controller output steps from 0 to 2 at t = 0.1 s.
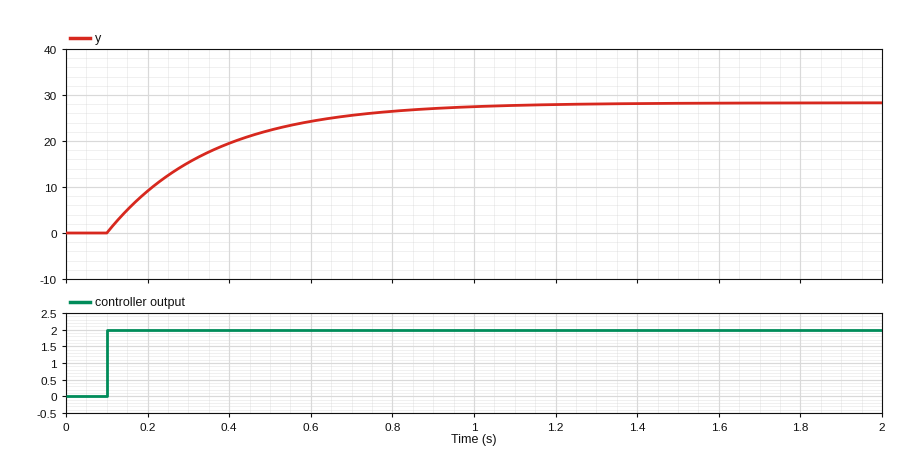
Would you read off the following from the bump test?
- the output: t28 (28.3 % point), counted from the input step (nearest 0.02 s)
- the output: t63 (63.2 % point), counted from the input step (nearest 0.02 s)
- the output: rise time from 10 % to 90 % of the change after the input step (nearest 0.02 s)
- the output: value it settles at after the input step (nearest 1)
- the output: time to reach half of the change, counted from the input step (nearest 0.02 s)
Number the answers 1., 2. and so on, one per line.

1. 0.08 s
2. 0.26 s
3. 0.56 s
4. 28
5. 0.18 s
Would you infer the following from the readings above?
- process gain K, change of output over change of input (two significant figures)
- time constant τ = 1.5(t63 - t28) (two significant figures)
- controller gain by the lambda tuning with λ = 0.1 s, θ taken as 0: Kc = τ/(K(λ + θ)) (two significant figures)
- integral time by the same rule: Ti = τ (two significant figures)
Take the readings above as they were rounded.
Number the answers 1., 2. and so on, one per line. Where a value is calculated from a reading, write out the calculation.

1. (28 - 0) / 2 = 14
2. 1.5 × (0.26 - 0.08) = 0.27 s
3. 0.27 / (14 × (0.1 + 0)) = 0.19
4. 0.27 s
